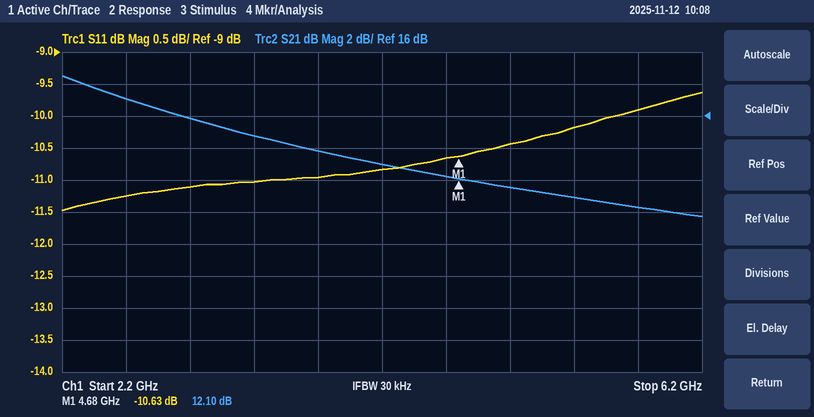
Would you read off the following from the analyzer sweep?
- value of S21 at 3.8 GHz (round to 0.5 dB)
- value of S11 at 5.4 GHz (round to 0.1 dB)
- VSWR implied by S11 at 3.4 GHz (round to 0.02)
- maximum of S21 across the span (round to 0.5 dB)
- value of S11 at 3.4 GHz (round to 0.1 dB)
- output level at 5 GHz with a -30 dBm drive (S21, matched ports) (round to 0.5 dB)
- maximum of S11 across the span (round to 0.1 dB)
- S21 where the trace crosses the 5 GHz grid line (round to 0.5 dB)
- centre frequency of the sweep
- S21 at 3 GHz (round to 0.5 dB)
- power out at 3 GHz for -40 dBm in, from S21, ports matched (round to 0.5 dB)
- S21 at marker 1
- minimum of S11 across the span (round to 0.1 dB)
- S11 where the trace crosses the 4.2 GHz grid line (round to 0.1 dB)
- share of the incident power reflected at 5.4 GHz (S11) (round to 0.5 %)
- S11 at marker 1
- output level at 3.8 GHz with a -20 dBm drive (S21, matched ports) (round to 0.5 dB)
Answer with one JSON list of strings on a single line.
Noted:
["14.0 dB", "-10.2 dB", "1.78", "18.5 dB", "-11.0 dB", "-18.5 dBm", "-9.6 dB", "11.5 dB", "4.2 GHz", "16.0 dB", "-24.0 dBm", "12.10 dB", "-11.5 dB", "-10.8 dB", "9.5 %", "-10.63 dB", "-6.0 dBm"]
